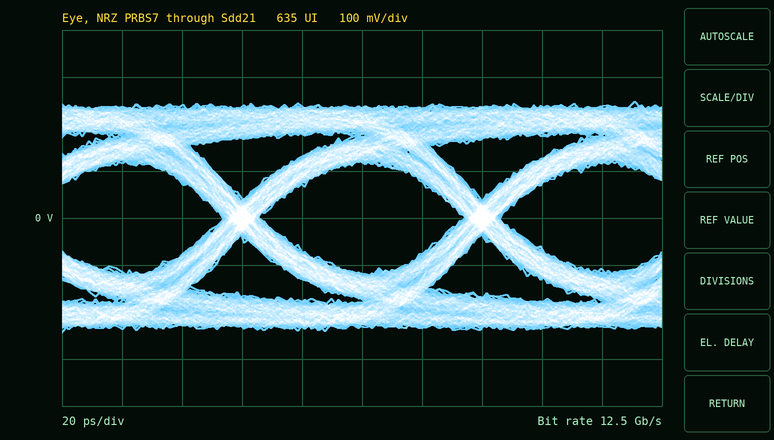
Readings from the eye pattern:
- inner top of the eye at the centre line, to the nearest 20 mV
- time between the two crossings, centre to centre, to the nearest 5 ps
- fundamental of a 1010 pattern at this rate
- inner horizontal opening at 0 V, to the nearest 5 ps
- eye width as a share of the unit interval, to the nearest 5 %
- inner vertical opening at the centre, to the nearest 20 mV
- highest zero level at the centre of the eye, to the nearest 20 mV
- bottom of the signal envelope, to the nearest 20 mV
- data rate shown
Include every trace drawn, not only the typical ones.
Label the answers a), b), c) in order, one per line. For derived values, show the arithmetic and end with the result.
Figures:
a) 120 mV
b) 80 ps
c) 6.25 GHz
d) 70 ps
e) 70 ps / 80 ps ≈ 87.5 %, so 85 % to the nearest 5 %
f) 240 mV
g) -120 mV
h) -240 mV
i) 12.5 Gb/s
